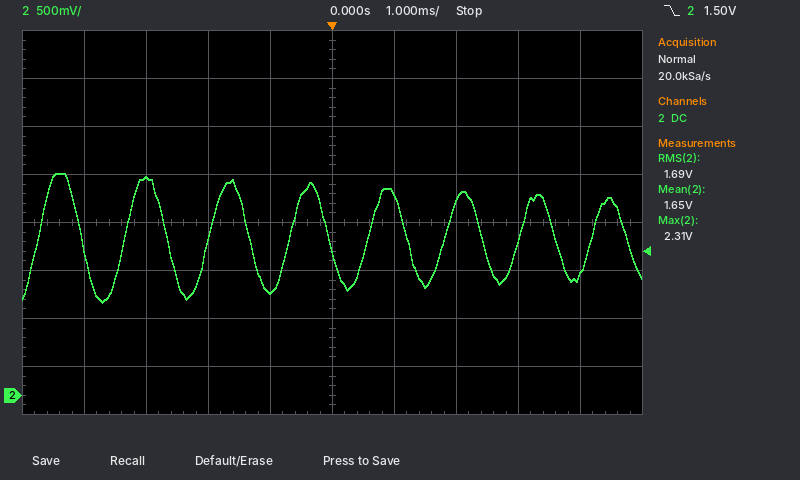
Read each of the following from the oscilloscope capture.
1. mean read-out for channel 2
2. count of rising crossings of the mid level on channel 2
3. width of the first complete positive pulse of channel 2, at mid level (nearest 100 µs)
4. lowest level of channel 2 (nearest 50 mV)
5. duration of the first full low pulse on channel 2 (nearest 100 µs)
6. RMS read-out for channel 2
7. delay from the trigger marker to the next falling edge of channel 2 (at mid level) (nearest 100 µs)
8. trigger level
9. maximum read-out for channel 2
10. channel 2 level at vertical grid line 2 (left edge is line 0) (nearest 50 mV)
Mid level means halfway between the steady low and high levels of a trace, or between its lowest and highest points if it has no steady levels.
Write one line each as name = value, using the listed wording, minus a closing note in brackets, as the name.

mean read-out for channel 2 = 1.65 V
count of rising crossings of the mid level on channel 2 = 8
width of the first complete positive pulse of channel 2, at mid level = 700 µs
lowest level of channel 2 = 950 mV
duration of the first full low pulse on channel 2 = 700 µs
RMS read-out for channel 2 = 1.69 V
delay from the trigger marker to the next falling edge of channel 2 (at mid level) = 1.2 ms
trigger level = 1.50 V
maximum read-out for channel 2 = 2.31 V
channel 2 level at vertical grid line 2 (left edge is line 0) = 2.25 V
